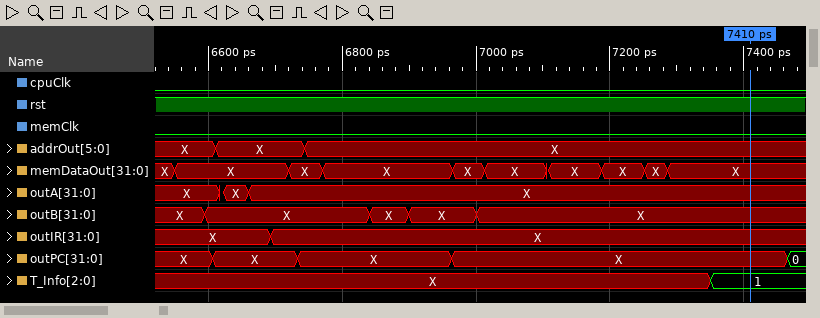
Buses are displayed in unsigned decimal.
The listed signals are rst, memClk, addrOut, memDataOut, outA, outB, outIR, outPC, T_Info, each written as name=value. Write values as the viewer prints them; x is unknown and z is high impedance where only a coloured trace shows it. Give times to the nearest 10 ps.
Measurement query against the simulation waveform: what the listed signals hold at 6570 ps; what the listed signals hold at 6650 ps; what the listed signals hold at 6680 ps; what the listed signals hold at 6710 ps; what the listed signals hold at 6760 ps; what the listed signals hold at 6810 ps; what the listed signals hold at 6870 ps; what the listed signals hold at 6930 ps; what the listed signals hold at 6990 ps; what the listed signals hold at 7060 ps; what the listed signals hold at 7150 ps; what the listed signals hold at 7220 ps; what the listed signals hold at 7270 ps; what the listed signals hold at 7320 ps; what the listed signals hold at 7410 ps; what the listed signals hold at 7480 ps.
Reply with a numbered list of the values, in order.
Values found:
1. rst=1, memClk=0, addrOut=X, memDataOut=X, outA=X, outB=X, outIR=X, outPC=X, T_Info=X
2. rst=1, memClk=0, addrOut=X, memDataOut=X, outA=X, outB=X, outIR=X, outPC=X, T_Info=X
3. rst=1, memClk=0, addrOut=X, memDataOut=X, outA=X, outB=X, outIR=X, outPC=X, T_Info=X
4. rst=1, memClk=0, addrOut=X, memDataOut=X, outA=X, outB=X, outIR=X, outPC=X, T_Info=X
5. rst=1, memClk=0, addrOut=X, memDataOut=X, outA=X, outB=X, outIR=X, outPC=X, T_Info=X
6. rst=1, memClk=0, addrOut=X, memDataOut=X, outA=X, outB=X, outIR=X, outPC=X, T_Info=X
7. rst=1, memClk=0, addrOut=X, memDataOut=X, outA=X, outB=X, outIR=X, outPC=X, T_Info=X
8. rst=1, memClk=0, addrOut=X, memDataOut=X, outA=X, outB=X, outIR=X, outPC=X, T_Info=X
9. rst=1, memClk=0, addrOut=X, memDataOut=X, outA=X, outB=X, outIR=X, outPC=X, T_Info=X
10. rst=1, memClk=0, addrOut=X, memDataOut=X, outA=X, outB=X, outIR=X, outPC=X, T_Info=X
11. rst=1, memClk=0, addrOut=X, memDataOut=X, outA=X, outB=X, outIR=X, outPC=X, T_Info=X
12. rst=1, memClk=0, addrOut=X, memDataOut=X, outA=X, outB=X, outIR=X, outPC=X, T_Info=X
13. rst=1, memClk=0, addrOut=X, memDataOut=X, outA=X, outB=X, outIR=X, outPC=X, T_Info=X
14. rst=1, memClk=0, addrOut=X, memDataOut=X, outA=X, outB=X, outIR=X, outPC=X, T_Info=X
15. rst=1, memClk=0, addrOut=X, memDataOut=X, outA=X, outB=X, outIR=X, outPC=X, T_Info=1
16. rst=1, memClk=0, addrOut=X, memDataOut=X, outA=X, outB=X, outIR=X, outPC=0, T_Info=1
